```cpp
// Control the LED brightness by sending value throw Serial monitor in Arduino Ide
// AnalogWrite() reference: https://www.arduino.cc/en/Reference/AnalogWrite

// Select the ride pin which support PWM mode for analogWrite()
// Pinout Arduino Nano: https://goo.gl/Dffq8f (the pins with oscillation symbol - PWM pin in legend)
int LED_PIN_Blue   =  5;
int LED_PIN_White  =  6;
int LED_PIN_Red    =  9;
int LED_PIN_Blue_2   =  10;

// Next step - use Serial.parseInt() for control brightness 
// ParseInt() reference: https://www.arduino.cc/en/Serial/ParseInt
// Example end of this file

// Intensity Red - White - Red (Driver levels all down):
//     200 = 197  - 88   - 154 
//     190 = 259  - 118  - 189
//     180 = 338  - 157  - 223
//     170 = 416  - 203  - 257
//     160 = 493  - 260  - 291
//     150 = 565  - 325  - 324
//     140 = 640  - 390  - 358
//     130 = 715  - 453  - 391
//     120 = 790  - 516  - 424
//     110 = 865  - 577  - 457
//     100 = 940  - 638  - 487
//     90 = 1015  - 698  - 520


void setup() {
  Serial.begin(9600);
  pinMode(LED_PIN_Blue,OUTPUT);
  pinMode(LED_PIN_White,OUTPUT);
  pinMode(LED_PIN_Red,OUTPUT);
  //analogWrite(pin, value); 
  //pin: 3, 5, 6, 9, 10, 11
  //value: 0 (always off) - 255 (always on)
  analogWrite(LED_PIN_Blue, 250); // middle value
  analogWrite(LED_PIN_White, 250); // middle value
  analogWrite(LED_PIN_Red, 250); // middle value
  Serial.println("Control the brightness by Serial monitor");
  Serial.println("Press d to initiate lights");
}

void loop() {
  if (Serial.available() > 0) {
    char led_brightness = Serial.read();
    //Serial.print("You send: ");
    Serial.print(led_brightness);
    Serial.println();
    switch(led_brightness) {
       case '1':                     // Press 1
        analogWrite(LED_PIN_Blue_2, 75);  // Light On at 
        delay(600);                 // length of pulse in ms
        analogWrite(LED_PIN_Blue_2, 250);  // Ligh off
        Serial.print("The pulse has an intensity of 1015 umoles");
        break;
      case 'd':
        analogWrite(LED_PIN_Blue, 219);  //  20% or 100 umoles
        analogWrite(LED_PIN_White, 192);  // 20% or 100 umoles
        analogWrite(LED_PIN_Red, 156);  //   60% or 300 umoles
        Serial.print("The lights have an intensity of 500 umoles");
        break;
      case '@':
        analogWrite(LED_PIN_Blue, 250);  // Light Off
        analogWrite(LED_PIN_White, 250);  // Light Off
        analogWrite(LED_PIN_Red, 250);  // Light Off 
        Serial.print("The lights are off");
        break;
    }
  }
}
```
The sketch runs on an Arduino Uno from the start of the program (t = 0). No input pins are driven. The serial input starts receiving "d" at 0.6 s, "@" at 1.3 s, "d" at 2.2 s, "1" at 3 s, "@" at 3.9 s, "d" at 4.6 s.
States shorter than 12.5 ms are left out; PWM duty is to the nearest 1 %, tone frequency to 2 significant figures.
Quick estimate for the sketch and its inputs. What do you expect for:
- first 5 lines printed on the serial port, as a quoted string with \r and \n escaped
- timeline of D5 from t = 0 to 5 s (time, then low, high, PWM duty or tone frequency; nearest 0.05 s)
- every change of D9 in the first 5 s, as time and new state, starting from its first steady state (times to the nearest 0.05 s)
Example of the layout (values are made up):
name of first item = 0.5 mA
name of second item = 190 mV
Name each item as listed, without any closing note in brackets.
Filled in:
first 5 lines printed on the serial port, as a quoted string with \r and \n escaped = "Control the brightness by Serial monitor\r\nPress d to initiate lights\r\nd\r\nThe lights have an intensity of 500 umoles@\r\nThe lights are offd\r\n"
timeline of D5 from t = 0 to 5 s = 0 s PWM 98 %; 0.6 s PWM 86 %; 1.3 s PWM 98 %; 2.2 s PWM 86 %; 3.9 s PWM 98 %; 4.6 s PWM 86 %
every change of D9 in the first 5 s, as time and new state, starting from its first steady state = 0 s PWM 98 %; 0.6 s PWM 61 %; 1.3 s PWM 98 %; 2.2 s PWM 61 %; 3.9 s PWM 98 %; 4.6 s PWM 61 %
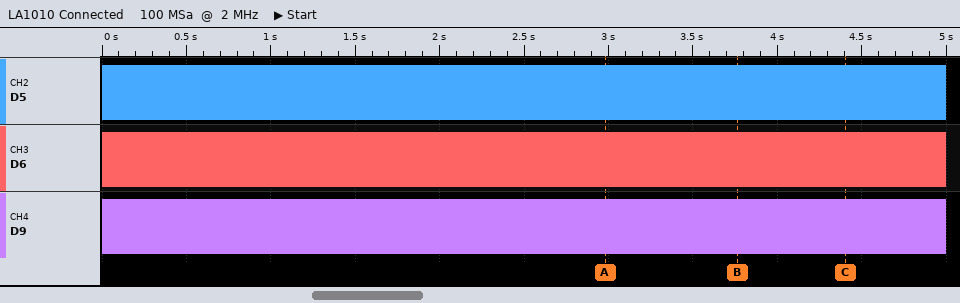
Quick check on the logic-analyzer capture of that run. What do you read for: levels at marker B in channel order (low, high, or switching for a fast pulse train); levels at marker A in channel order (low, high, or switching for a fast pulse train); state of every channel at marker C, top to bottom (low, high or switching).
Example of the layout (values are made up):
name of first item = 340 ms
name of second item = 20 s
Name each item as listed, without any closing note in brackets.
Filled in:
levels at marker B in channel order = D5 switching, D6 switching, D9 switching
levels at marker A in channel order = D5 switching, D6 switching, D9 switching
state of every channel at marker C, top to bottom = D5 switching, D6 switching, D9 switching
